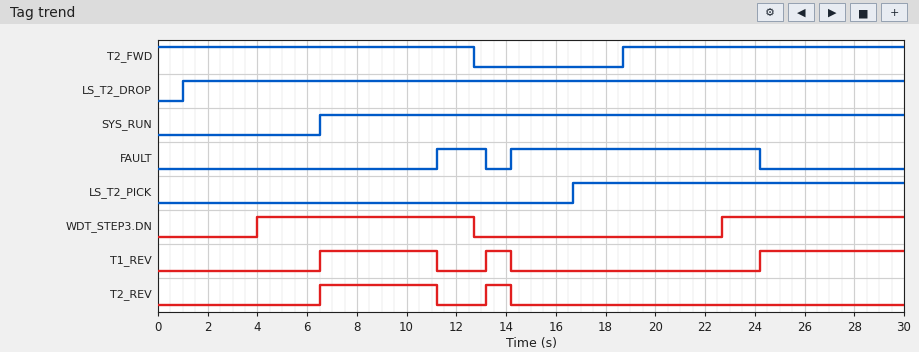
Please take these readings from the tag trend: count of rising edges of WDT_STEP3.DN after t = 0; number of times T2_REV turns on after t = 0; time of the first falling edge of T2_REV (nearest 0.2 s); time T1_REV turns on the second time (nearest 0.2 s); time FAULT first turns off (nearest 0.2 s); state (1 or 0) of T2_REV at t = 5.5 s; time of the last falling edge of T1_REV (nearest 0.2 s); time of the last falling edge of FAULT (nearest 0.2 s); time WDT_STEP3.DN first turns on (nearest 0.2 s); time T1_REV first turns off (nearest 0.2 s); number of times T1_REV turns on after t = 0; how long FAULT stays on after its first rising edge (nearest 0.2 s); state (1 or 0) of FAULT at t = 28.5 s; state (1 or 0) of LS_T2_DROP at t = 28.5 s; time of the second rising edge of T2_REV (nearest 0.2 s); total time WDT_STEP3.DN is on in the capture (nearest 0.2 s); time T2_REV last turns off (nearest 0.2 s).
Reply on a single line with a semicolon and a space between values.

2; 2; 11.2 s; 13.2 s; 13.2 s; 0; 14.2 s; 24.2 s; 4.0 s; 11.2 s; 3; 2.0 s; 0; 1; 13.2 s; 16.0 s; 14.2 s
